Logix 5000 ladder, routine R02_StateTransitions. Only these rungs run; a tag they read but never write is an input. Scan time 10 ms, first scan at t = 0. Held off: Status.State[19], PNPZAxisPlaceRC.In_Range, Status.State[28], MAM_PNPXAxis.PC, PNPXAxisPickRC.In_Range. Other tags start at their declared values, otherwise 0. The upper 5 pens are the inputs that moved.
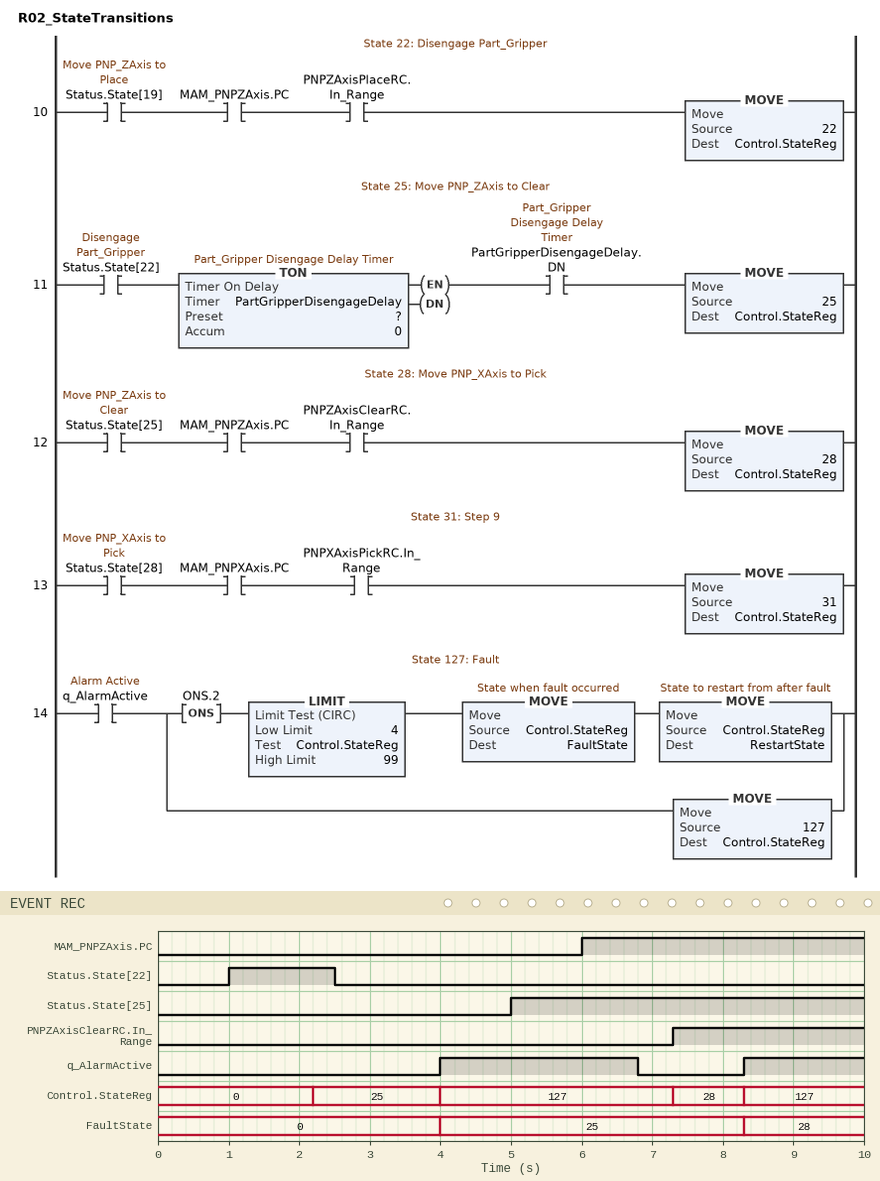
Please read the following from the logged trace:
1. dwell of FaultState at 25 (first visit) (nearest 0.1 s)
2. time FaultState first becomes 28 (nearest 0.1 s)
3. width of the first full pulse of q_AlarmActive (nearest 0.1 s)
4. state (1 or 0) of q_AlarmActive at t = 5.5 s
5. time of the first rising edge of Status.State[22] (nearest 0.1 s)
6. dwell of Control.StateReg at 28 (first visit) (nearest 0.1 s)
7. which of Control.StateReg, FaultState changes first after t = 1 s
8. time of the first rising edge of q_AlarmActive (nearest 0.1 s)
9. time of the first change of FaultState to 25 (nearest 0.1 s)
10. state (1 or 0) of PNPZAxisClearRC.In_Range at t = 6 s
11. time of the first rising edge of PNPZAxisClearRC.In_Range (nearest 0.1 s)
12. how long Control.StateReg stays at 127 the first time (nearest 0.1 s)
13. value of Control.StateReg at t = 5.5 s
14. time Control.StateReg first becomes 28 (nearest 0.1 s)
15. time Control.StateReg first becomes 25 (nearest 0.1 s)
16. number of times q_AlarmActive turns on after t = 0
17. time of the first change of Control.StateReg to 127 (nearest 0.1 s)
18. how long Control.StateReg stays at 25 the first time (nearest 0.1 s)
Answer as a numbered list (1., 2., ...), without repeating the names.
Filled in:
1. 4.3 s
2. 8.3 s
3. 2.8 s
4. 1
5. 1.0 s
6. 1.0 s
7. Control.StateReg
8. 4.0 s
9. 4.0 s
10. 0
11. 7.3 s
12. 3.3 s
13. 127
14. 7.3 s
15. 2.2 s
16. 2
17. 4.0 s
18. 1.8 s
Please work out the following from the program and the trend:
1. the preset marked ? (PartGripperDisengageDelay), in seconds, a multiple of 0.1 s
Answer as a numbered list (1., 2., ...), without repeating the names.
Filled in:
1. 1.2 s
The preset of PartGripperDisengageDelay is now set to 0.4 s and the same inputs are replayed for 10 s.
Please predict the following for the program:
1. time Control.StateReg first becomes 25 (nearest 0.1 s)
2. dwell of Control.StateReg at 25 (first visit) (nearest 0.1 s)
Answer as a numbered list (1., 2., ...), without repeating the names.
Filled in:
1. 1.4 s
2. 2.6 s
